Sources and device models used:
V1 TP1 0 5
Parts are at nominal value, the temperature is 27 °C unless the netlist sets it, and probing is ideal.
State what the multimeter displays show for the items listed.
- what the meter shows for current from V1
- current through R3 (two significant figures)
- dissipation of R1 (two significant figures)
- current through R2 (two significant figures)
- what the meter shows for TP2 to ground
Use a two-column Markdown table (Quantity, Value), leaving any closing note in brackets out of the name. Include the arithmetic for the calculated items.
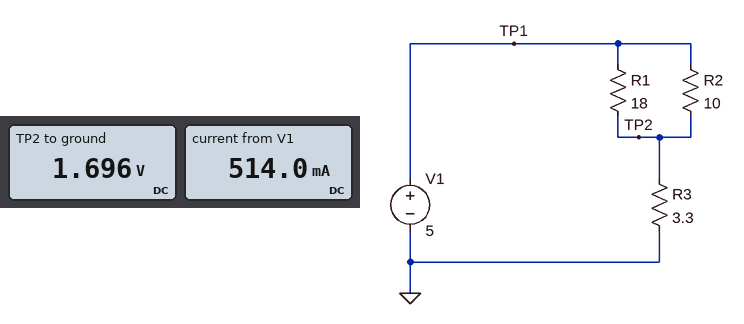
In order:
| Quantity | Value |
|---|---|
| what the meter shows for current from V1 | 514.0 mA |
| current through R3 | (1.696 V) / 3.3 Ω = 510 mA |
| dissipation of R1 | (5 V - 1.696 V)^2 / 18 Ω = 610 mW |
| current through R2 | (5 V - 1.696 V) / 10 Ω = 330 mA |
| what the meter shows for TP2 to ground | 1.696 V |
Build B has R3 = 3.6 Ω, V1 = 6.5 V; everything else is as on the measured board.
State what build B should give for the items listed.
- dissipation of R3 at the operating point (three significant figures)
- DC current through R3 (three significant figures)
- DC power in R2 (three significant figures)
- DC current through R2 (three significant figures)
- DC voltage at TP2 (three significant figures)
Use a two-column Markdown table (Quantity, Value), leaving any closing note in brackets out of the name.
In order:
| Quantity | Value |
|---|---|
| dissipation of R3 at the operating point | 1.51 W |
| DC current through R3 | 648 mA |
| DC power in R2 | 1.74 W |
| DC current through R2 | 417 mA |
| DC voltage at TP2 | 2.33 V |
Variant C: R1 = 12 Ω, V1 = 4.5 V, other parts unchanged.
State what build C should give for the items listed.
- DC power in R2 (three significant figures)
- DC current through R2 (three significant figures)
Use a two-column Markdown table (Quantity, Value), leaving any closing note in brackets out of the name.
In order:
| Quantity | Value |
|---|---|
| DC power in R2 | 786 mW |
| DC current through R2 | 280 mA |
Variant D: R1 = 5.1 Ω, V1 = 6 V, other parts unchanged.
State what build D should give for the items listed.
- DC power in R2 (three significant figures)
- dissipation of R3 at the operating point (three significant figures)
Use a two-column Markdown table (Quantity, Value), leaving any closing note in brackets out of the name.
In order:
| Quantity | Value |
|---|---|
| DC power in R2 | 921 mW |
| dissipation of R3 at the operating point | 2.66 W |
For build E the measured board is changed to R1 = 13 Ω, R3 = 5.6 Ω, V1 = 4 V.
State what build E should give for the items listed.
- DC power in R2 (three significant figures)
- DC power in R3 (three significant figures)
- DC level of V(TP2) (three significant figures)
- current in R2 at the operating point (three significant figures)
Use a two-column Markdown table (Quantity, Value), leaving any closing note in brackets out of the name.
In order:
| Quantity | Value |
|---|---|
| DC power in R2 | 404 mW |
| DC power in R3 | 708 mW |
| DC level of V(TP2) | 1.99 V |
| current in R2 at the operating point | 201 mA |
